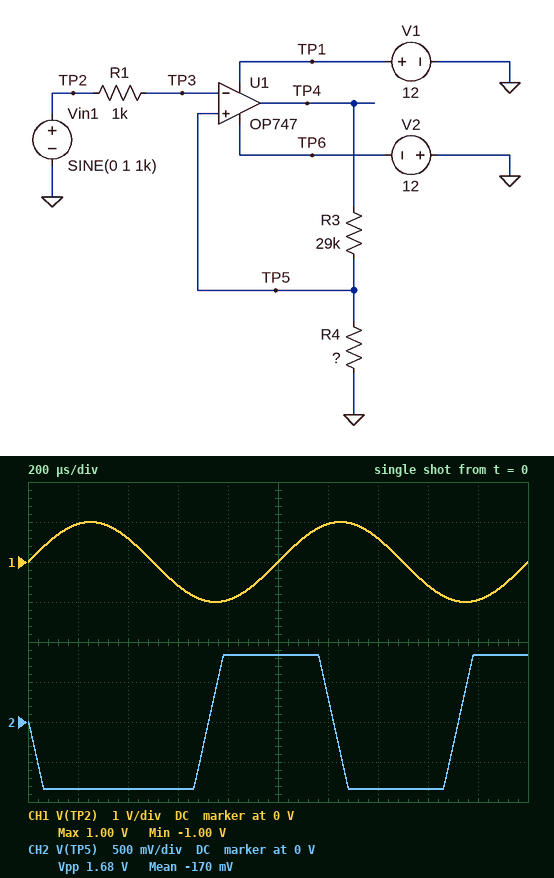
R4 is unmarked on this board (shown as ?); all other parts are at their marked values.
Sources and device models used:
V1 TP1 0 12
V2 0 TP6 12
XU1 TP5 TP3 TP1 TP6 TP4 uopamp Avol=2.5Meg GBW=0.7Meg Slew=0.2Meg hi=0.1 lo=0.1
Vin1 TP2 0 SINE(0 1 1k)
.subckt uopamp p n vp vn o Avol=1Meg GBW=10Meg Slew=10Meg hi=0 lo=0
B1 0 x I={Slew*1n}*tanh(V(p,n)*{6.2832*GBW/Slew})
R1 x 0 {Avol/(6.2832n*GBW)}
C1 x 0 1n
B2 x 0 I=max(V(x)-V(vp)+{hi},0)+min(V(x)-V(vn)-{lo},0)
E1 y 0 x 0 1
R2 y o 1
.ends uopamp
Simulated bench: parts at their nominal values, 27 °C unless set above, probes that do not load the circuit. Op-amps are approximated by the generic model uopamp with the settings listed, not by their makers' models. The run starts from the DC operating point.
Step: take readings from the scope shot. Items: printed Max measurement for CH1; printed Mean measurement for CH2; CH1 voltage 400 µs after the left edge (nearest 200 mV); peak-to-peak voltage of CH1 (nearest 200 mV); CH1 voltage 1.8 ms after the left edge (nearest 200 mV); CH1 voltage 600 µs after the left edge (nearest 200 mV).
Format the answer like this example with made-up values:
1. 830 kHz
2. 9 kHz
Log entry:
1. 1.00 V
2. -170 mV
3. 600 mV
4. 2.0 V
5. -1.0 V
6. -600 mV
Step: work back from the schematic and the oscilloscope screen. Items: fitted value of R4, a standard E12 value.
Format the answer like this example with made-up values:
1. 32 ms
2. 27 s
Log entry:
1. 2.2 kΩ
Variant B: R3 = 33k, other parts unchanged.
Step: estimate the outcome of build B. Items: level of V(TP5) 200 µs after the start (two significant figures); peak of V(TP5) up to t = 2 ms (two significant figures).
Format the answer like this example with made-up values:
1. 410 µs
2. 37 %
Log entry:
1. -740 mV
2. 740 mV
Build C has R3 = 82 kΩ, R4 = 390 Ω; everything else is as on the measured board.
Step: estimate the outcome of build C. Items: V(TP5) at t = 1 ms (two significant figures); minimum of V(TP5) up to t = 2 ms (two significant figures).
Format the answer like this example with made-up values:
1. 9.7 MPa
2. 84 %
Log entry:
1. 56 mV
2. -56 mV
